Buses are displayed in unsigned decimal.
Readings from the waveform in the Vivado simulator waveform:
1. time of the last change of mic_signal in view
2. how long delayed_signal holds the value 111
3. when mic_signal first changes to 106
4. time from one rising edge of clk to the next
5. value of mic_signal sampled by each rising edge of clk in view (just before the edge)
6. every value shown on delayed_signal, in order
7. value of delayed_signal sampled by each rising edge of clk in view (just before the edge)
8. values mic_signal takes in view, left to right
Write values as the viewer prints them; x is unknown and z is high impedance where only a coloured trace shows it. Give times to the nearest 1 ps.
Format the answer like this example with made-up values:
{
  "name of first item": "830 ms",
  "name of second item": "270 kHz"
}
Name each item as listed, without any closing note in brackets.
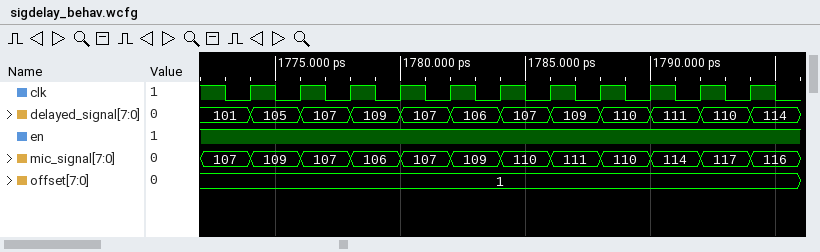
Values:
{
  "time of the last change of mic_signal in view": "1794 ps",
  "how long delayed_signal holds the value 111": "2 ps",
  "when mic_signal first changes to 106": "1778 ps",
  "time from one rising edge of clk to the next": "2 ps",
  "value of mic_signal sampled by each rising edge of clk in view": "107, 109, 107, 106, 107, 109, 110, 111, 110, 114, 117",
  "every value shown on delayed_signal, in order": "101, 105, 107, 109, 107, 106, 107, 109, 110, 111, 110, 114",
  "value of delayed_signal sampled by each rising edge of clk in view": "101, 105, 107, 109, 107, 106, 107, 109, 110, 111, 110",
  "values mic_signal takes in view, left to right": "107, 109, 107, 106, 107, 109, 110, 111, 110, 114, 117, 116"
}
